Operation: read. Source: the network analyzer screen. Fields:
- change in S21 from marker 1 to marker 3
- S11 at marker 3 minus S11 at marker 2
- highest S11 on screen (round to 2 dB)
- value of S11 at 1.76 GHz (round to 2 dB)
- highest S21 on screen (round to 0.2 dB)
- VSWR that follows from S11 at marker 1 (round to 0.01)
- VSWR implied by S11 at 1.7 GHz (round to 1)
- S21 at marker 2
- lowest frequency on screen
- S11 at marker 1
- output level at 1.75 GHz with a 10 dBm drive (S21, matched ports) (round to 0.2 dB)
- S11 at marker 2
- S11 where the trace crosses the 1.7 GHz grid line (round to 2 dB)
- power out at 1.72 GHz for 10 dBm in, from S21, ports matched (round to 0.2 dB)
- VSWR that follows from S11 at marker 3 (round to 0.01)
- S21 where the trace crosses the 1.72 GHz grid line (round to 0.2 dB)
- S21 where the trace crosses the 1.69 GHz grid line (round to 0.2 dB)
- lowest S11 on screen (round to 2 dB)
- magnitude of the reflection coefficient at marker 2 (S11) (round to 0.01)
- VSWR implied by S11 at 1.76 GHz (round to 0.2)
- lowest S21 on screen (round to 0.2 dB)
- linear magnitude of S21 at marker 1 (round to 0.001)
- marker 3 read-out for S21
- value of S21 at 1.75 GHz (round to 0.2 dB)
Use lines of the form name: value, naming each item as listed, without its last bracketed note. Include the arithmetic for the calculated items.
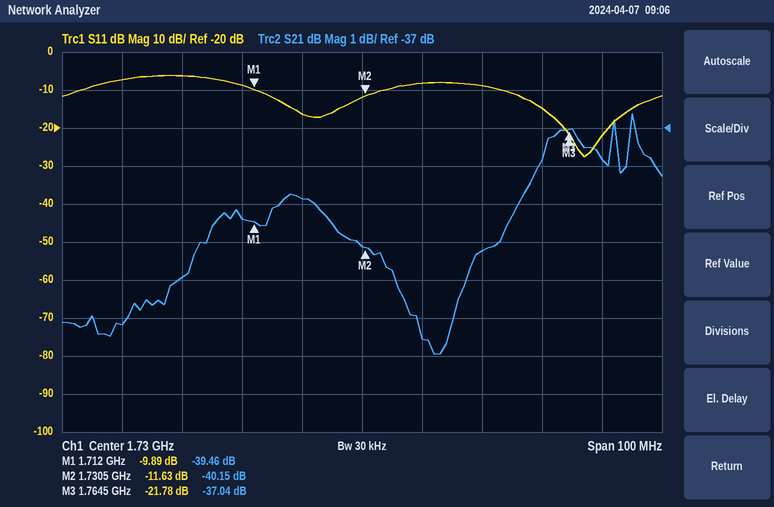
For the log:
change in S21 from marker 1 to marker 3: -37.04 − (-39.46) = 2.42 dB
S11 at marker 3 minus S11 at marker 2: -21.78 − (-11.63) = -10.15 dB
highest S11 on screen: -6 dB
value of S11 at 1.76 GHz: -14 dB
highest S21 on screen: -36.6 dB
VSWR that follows from S11 at marker 1: (1 + 0.3203)/(1 − 0.3203) ≈ 1.94
VSWR implied by S11 at 1.7 GHz: |Γ| = 10^(-6/20) = 0.5012; VSWR = (1 + 0.5012)/(1 − 0.5012) ≈ 3
S21 at marker 2: -40.15 dB
lowest frequency on screen: 1.68 GHz
S11 at marker 1: -9.89 dB
output level at 1.75 GHz with a 10 dBm drive (S21, matched ports): 10 dBm + (-40.2 dB) = -30.2 dBm
S11 at marker 2: -11.63 dB
S11 where the trace crosses the 1.7 GHz grid line: -6 dB
power out at 1.72 GHz for 10 dBm in, from S21, ports matched: 10 dBm + (-38.8 dB) = -28.8 dBm
VSWR that follows from S11 at marker 3: (1 + 0.0815)/(1 − 0.0815) ≈ 1.18
S21 where the trace crosses the 1.72 GHz grid line: -38.8 dB
S21 where the trace crosses the 1.69 GHz grid line: -42.2 dB
lowest S11 on screen: -28 dB
magnitude of the reflection coefficient at marker 2 (S11): 10^(-11.63/20) ≈ 0.26
VSWR implied by S11 at 1.76 GHz: |Γ| = 10^(-14/20) = 0.1995; VSWR = (1 + 0.1995)/(1 − 0.1995) ≈ 1.50, so 1.4 to the nearest 0.2
lowest S21 on screen: -43.0 dB
linear magnitude of S21 at marker 1: 10^(-39.46/20) ≈ 0.011
marker 3 read-out for S21: -37.04 dB
value of S21 at 1.75 GHz: -40.2 dB
